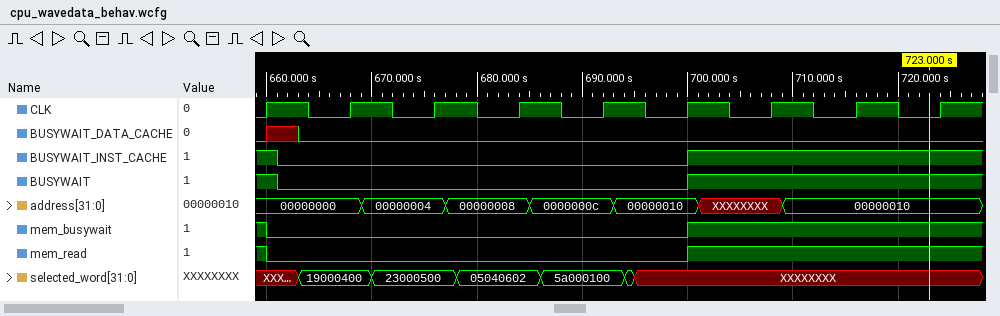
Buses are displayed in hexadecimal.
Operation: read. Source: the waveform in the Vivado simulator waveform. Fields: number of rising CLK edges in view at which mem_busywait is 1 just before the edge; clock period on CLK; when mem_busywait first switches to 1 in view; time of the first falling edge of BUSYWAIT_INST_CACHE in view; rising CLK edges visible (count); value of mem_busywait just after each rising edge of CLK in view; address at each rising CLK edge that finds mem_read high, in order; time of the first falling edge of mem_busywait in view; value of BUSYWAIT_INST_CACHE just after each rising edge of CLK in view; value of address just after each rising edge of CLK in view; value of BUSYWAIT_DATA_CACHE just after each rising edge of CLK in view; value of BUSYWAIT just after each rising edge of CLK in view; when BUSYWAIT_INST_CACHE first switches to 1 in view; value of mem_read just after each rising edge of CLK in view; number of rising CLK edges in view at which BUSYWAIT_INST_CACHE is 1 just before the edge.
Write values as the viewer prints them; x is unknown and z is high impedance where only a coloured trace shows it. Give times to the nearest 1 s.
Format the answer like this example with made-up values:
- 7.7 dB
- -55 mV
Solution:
- 4
- 8 s
- 700 s
- 661 s
- 9
- 0 0 0 0 0 1 1 1 1
- 00000000, XXXXXXXX, 00000010, 00000010
- 660 s
- 1 0 0 0 0 1 1 1 1
- 00000000, 00000000, 00000004, 00000008, 0000000c, 00000010, XXXXXXXX, 00000010, 00000010
- x 0 0 0 0 0 0 0 0
- 1 0 0 0 0 1 1 1 1
- 700 s
- 0 0 0 0 0 1 1 1 1
- 4
